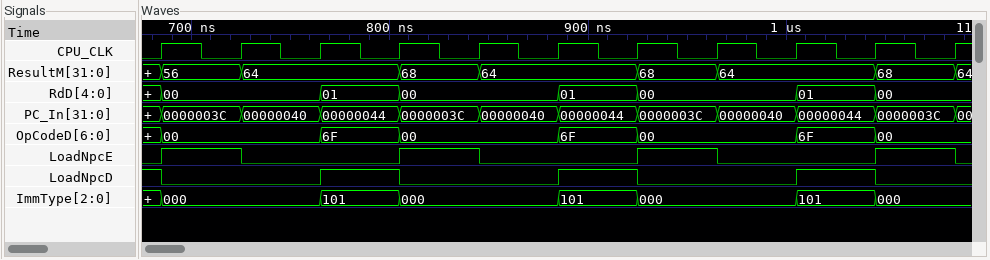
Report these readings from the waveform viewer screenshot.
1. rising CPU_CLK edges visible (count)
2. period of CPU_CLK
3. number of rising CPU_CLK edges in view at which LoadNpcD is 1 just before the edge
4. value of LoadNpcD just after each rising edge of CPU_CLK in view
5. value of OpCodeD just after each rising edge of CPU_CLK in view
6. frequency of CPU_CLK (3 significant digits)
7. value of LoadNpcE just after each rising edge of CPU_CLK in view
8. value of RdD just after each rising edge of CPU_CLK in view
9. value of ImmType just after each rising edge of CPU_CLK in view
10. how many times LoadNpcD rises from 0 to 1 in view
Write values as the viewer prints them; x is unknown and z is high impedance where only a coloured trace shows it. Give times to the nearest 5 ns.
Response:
11
40 ns
4
0 0 1 0 0 1 0 0 1 0 0
00, 00, 6F, 00, 00, 6F, 00, 00, 6F, 00, 00
25.0 MHz
1 0 0 1 0 0 1 0 0 1 0
00, 00, 01, 00, 00, 01, 00, 00, 01, 00, 00
000, 000, 101, 000, 000, 101, 000, 000, 101, 000, 000
3
